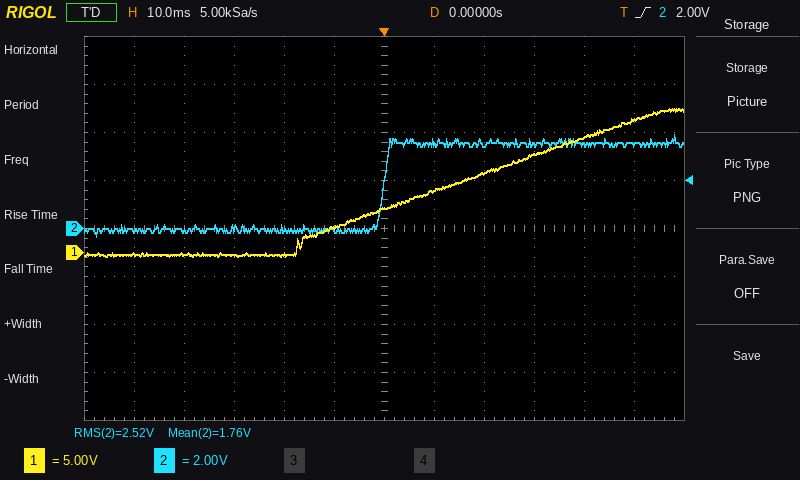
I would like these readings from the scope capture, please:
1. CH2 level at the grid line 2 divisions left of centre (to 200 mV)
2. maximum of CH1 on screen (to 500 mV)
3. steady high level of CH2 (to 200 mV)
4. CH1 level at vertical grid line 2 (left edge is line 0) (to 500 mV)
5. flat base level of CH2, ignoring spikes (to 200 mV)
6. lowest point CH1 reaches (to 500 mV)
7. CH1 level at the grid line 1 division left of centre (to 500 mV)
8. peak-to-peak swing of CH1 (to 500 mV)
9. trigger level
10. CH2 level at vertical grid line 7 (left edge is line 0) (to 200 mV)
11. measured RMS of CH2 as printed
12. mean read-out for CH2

0.0 V
15.0 V
3.6 V
0.0 V
0.0 V
-500 mV
2.5 V
15.5 V
2.00 V
3.6 V
2.52 V
1.76 V
